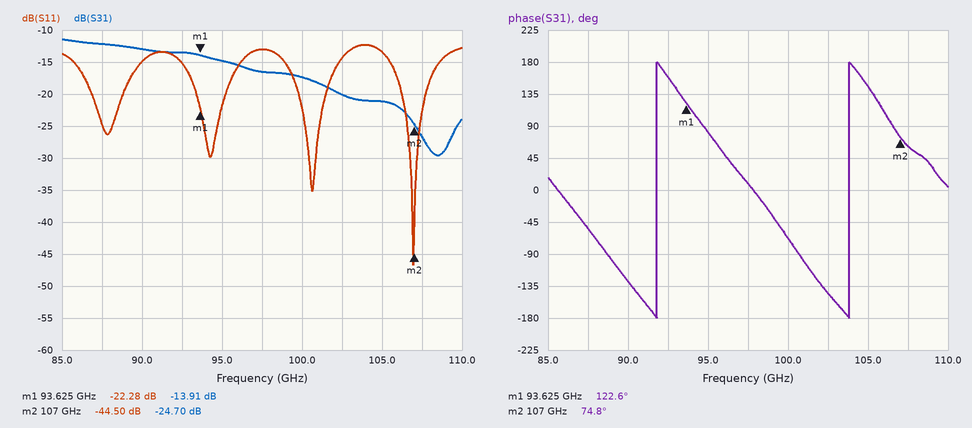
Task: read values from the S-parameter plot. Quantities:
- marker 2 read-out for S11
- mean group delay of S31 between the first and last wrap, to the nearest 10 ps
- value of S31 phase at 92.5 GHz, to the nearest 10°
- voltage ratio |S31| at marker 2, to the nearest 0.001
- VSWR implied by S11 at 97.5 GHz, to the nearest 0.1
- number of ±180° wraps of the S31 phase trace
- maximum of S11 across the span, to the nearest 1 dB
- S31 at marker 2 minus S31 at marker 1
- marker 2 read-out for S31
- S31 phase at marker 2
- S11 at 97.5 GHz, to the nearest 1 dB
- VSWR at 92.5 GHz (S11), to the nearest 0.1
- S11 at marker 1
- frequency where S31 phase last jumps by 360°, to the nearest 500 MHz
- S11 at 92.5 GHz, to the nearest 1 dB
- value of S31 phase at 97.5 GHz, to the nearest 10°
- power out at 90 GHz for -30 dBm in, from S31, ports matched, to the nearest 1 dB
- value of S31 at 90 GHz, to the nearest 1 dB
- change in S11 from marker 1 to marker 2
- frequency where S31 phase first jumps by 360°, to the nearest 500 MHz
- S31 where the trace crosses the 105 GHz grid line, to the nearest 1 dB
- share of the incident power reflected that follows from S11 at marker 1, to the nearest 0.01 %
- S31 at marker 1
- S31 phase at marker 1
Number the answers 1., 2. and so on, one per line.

1. -44.50 dB
2. 80 ps
3. 160°
4. 0.058
5. 1.6
6. 2
7. -12 dB
8. -10.79 dB
9. -24.70 dB
10. 74.8°
11. -13 dB
12. 1.4
13. -22.28 dB
14. 104.0 GHz
15. -15 dB
16. 10°
17. -43 dBm
18. -13 dB
19. -22.22 dB
20. 92.0 GHz
21. -21 dB
22. 0.59 %
23. -13.91 dB
24. 122.6°
